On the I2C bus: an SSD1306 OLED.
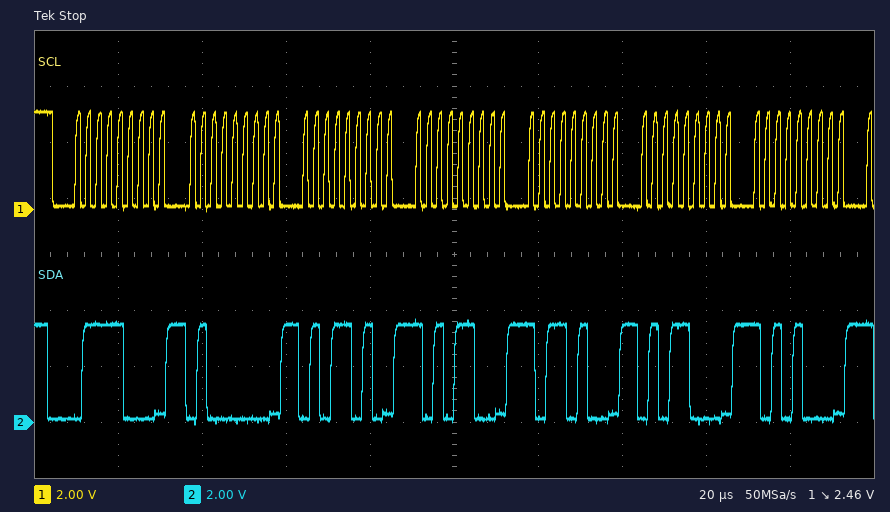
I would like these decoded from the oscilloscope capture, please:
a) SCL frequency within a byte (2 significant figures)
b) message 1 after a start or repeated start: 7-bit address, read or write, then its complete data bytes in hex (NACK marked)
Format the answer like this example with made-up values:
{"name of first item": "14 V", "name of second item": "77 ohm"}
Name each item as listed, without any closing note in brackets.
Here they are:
{"SCL frequency within a byte": "400 kHz", "message 1 after a start or repeated start: 7-bit address, read or write, then its complete data bytes in hex": "0x3C write: 40 5A AC B4 58 A8"}
